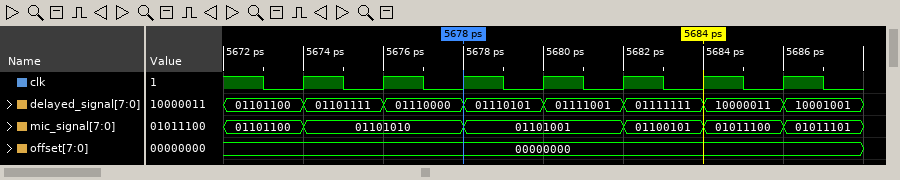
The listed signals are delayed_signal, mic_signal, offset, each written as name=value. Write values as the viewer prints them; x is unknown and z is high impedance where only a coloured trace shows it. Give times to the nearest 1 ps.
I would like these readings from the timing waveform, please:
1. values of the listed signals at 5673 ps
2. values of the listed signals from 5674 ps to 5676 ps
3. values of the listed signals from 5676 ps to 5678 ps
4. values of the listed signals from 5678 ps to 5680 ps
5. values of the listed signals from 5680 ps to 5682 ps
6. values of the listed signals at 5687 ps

delayed_signal=01101100, mic_signal=01101100, offset=00000000
delayed_signal=01101111, mic_signal=01101010, offset=00000000
delayed_signal=01110000, mic_signal=01101010, offset=00000000
delayed_signal=01110101, mic_signal=01101001, offset=00000000
delayed_signal=01111001, mic_signal=01101001, offset=00000000
delayed_signal=10001001, mic_signal=01011101, offset=00000000
